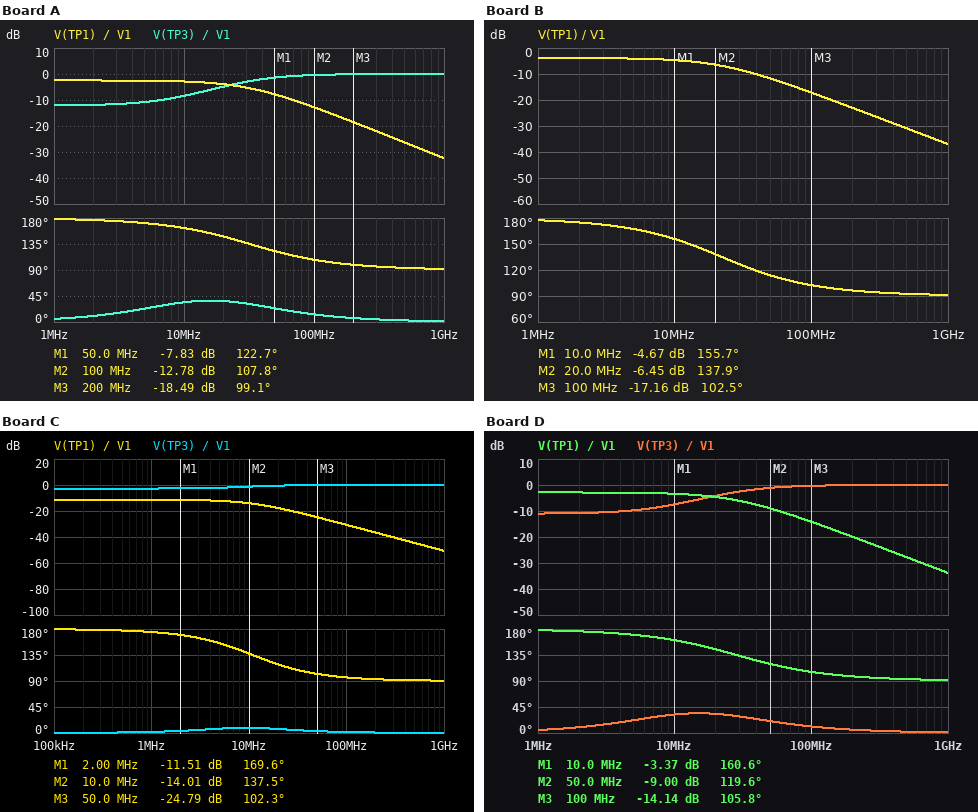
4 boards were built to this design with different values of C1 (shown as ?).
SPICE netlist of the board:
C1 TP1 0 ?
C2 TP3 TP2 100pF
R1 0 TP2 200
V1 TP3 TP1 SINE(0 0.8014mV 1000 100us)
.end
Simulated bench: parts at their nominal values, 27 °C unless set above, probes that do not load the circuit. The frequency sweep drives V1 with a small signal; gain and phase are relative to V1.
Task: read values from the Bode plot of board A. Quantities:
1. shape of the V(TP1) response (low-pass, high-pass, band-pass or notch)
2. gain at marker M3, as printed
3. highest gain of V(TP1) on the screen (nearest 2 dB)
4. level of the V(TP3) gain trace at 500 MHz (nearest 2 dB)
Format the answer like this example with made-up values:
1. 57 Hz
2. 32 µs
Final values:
1. low-pass
2. -18.49 dB
3. -2 dB
4. 0 dB
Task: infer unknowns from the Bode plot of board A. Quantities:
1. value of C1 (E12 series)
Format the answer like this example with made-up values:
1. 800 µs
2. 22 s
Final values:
1. 33 pF
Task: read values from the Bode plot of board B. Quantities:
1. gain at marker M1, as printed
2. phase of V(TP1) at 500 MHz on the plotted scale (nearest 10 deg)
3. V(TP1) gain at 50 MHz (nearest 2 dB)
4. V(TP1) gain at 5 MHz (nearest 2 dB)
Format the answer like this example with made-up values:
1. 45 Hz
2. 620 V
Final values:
1. -4.67 dB
2. 90 deg
3. -12 dB
4. -4 dB
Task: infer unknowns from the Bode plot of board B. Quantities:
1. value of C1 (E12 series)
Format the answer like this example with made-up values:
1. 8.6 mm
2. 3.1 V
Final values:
1. 56 pF
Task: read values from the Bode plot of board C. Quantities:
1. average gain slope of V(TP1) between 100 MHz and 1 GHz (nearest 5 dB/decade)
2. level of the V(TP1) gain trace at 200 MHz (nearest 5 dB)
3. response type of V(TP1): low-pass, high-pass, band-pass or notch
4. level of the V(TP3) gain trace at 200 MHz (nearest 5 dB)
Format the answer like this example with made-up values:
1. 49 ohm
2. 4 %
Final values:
1. -20 dB/decade
2. -35 dB
3. low-pass
4. 0 dB
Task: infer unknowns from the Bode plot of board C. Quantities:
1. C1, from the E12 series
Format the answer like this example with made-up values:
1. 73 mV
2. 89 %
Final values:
1. 270 pF
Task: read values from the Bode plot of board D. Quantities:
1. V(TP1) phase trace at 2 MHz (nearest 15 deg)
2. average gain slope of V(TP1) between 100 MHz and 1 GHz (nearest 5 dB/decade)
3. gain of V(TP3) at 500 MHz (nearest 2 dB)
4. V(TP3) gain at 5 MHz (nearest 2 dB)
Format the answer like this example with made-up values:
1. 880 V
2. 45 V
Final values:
1. 180 deg
2. -20 dB/decade
3. 0 dB
4. -10 dB
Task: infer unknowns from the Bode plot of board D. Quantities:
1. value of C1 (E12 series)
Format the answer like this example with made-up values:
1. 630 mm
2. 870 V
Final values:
1. 39 pF
